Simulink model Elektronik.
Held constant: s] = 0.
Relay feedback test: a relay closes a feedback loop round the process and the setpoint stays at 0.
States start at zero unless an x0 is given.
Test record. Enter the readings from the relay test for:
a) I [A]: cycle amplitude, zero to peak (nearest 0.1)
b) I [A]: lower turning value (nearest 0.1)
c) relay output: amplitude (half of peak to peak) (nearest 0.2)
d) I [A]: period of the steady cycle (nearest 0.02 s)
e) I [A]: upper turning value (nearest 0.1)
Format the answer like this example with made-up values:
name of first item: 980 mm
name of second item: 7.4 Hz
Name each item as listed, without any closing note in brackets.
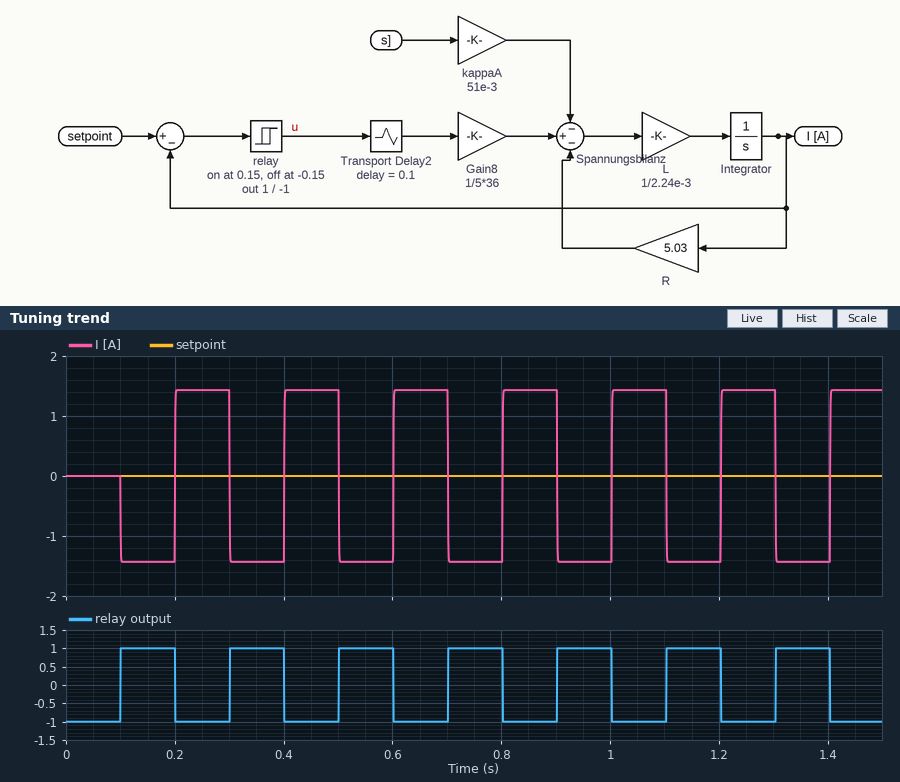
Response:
I [A]: cycle amplitude, zero to peak: 1.4
I [A]: lower turning value: -1.4
relay output: amplitude (half of peak to peak): 1.0
I [A]: period of the steady cycle: 0.20 s
I [A]: upper turning value: 1.4
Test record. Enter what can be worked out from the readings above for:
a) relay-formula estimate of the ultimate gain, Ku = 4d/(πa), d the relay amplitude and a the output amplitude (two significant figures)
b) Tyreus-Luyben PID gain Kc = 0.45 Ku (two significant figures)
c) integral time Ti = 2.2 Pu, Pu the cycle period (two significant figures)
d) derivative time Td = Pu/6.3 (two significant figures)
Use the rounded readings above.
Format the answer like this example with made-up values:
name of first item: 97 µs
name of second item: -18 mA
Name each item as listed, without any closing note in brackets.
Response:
relay-formula estimate of the ultimate gain, Ku = 4d/(πa), d the relay amplitude and a the output amplitude: 0.91
Tyreus-Luyben PID gain Kc = 0.45 Ku: 0.41
integral time Ti = 2.2 Pu, Pu the cycle period: 0.44 s
derivative time Td = Pu/6.3: 0.032 s
